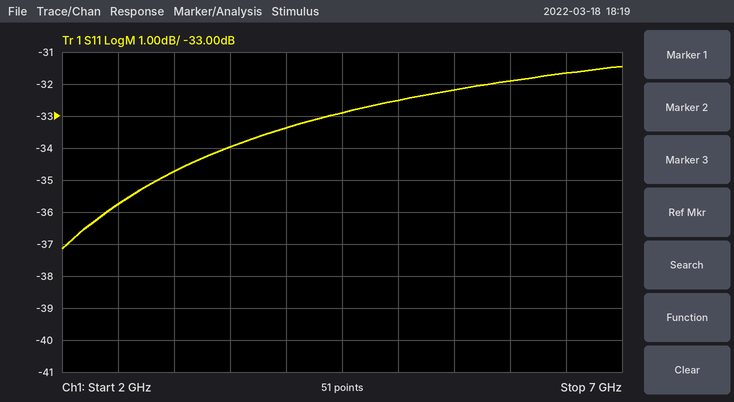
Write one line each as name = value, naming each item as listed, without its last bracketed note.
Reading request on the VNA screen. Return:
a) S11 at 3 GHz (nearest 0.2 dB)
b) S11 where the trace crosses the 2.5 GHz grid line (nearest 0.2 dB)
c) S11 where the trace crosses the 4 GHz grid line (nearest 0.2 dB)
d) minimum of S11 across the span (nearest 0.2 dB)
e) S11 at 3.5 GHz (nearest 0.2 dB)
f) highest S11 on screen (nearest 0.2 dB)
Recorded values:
S11 at 3 GHz = -34.8 dB
S11 where the trace crosses the 2.5 GHz grid line = -35.8 dB
S11 where the trace crosses the 4 GHz grid line = -33.4 dB
minimum of S11 across the span = -37.2 dB
S11 at 3.5 GHz = -34.0 dB
highest S11 on screen = -31.4 dB
